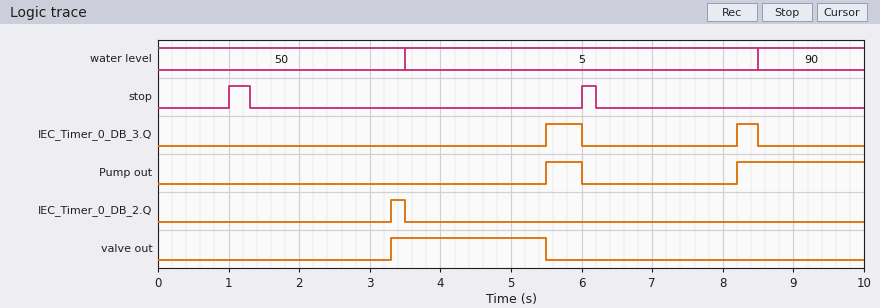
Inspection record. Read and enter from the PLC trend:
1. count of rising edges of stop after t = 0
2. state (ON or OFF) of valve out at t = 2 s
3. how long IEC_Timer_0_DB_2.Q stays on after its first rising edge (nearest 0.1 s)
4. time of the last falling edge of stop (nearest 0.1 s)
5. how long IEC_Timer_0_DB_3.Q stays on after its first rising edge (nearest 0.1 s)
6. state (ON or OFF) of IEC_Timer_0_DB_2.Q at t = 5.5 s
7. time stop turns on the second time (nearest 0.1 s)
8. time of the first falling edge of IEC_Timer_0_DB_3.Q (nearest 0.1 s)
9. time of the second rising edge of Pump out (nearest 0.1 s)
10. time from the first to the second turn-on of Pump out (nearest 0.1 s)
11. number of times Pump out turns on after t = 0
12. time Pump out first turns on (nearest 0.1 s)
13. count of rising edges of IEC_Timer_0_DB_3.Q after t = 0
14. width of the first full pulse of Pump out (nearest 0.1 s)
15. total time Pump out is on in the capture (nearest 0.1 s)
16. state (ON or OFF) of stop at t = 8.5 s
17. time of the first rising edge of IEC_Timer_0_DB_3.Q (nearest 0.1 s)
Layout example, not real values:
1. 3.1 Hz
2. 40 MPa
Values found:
1. 2
2. OFF
3. 0.2 s
4. 6.2 s
5. 0.5 s
6. OFF
7. 6.0 s
8. 6.0 s
9. 8.2 s
10. 2.7 s
11. 2
12. 5.5 s
13. 2
14. 0.5 s
15. 2.3 s
16. OFF
17. 5.5 s
